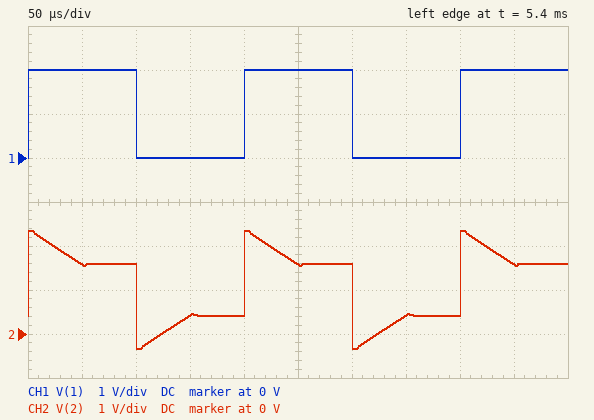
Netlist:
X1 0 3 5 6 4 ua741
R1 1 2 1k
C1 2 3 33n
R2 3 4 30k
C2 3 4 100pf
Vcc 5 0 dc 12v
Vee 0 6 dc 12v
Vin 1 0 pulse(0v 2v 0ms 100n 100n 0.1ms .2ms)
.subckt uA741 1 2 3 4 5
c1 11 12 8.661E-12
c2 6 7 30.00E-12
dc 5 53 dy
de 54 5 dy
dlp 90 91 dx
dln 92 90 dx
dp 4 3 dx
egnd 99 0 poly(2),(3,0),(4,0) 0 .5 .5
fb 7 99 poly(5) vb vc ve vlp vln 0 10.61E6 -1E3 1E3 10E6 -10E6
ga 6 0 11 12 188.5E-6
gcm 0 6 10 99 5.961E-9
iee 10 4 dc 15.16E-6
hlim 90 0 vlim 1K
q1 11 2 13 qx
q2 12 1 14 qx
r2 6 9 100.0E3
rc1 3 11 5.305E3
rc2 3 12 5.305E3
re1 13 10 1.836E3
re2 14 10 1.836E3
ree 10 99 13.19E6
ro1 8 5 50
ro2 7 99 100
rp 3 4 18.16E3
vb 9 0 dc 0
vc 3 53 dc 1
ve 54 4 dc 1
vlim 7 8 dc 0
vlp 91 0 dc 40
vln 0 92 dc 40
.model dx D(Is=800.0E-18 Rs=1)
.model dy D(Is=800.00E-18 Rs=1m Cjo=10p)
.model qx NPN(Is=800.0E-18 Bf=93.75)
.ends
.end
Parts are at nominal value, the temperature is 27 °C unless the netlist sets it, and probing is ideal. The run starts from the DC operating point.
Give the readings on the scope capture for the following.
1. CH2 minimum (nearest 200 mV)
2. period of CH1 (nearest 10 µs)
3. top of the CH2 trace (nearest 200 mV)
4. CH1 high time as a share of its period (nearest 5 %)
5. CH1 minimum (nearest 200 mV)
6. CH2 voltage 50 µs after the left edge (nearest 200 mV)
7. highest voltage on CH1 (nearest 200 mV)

-400 mV
200 µs
2.4 V
50 %
0 V
1.6 V
2.0 V
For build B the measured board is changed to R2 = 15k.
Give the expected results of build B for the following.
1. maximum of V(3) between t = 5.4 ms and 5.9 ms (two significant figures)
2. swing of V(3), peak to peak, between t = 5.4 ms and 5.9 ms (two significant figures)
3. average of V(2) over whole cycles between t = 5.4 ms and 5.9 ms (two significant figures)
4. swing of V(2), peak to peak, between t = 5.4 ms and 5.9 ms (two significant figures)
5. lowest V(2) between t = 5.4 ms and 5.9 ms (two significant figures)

1.8 V
3.7 V
1.0 V
2.0 V
-20 mV
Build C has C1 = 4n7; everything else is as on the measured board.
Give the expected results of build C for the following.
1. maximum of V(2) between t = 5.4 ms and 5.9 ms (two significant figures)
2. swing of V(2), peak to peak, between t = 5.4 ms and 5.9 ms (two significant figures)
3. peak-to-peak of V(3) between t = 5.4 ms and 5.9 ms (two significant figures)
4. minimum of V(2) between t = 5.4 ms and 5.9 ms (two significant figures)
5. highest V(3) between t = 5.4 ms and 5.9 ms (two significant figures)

2.2 V
2.3 V
3.7 V
-170 mV
1.8 V
